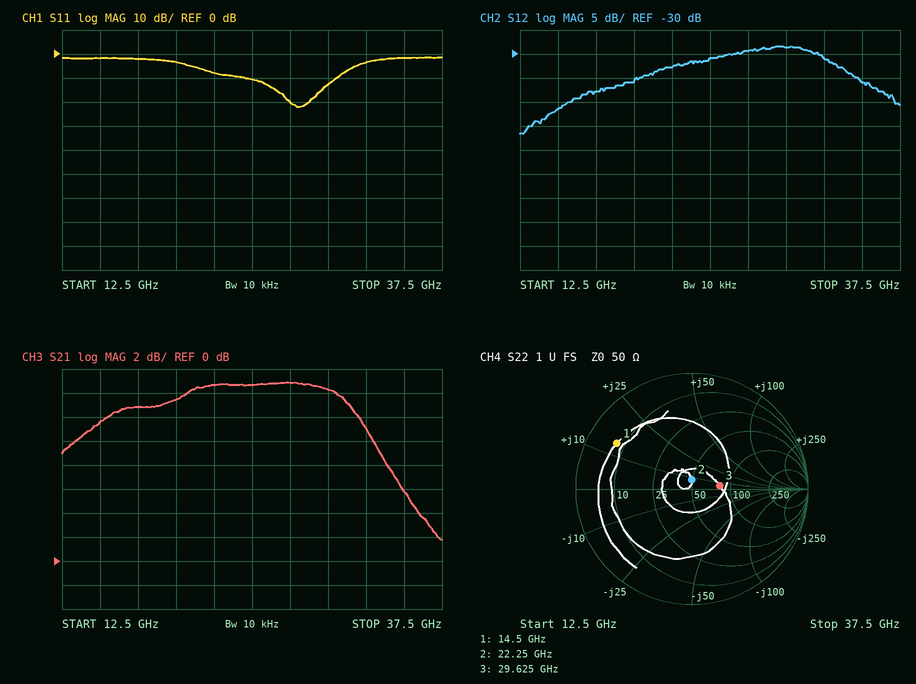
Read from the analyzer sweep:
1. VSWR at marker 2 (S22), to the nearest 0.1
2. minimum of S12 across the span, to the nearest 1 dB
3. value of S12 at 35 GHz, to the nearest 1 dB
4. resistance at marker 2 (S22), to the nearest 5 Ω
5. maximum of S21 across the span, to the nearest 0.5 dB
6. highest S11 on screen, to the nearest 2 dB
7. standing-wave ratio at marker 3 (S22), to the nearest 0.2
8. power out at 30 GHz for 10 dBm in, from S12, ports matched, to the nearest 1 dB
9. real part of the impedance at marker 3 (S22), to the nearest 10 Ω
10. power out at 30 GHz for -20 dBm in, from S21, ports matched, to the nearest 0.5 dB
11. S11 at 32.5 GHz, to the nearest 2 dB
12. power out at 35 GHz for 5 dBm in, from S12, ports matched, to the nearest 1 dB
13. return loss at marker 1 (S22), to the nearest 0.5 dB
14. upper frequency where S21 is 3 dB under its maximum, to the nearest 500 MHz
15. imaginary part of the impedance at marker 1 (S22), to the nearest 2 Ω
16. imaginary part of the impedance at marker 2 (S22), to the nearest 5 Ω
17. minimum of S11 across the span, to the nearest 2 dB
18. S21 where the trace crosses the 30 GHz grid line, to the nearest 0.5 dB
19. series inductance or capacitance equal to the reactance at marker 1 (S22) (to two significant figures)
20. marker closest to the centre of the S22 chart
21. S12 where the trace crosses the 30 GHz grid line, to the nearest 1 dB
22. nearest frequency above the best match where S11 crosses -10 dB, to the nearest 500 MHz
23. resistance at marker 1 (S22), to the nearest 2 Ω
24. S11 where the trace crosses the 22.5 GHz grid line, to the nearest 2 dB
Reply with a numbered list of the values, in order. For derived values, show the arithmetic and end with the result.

1. 1.2
2. -47 dB
3. -36 dB
4. 50 Ω
5. 15.0 dB
6. -2 dB
7. 1.6
8. 10 dBm + (-29 dB) = -19 dBm
9. 80 Ω
10. -20 dBm + (14.5 dB) = -5.5 dBm
11. -4 dB
12. 5 dBm + (-36 dB) = -31 dBm
13. 2.5 dB
14. 32.0 GHz
15. +14 Ω
16. +10 Ω
17. -22 dB
18. 14.5 dB
19. L = 14 Ω/(2π × 14.5 GHz) ≈ 154 pH, so 150 pH to two significant figures
20. marker 2
21. -29 dB
22. 30.5 GHz
23. 8 Ω
24. -8 dB
